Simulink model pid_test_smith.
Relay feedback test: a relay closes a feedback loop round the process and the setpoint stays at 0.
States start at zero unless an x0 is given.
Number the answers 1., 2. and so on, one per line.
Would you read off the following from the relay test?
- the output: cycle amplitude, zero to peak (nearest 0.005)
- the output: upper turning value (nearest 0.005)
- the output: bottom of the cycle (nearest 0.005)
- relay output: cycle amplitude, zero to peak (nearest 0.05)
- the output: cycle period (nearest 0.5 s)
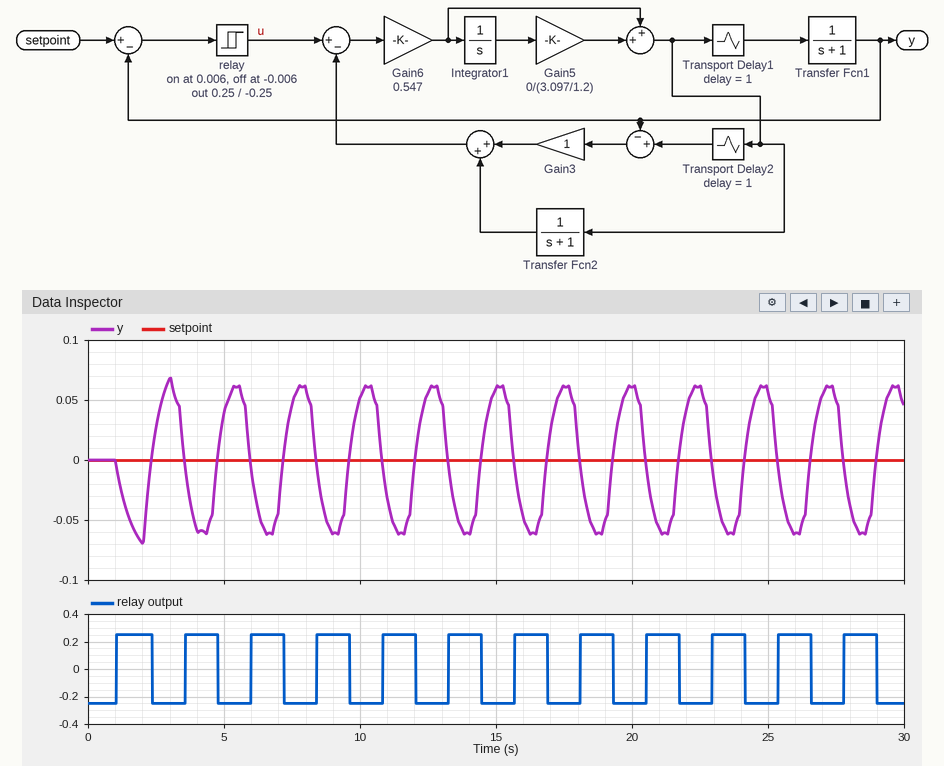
1. 0.060
2. 0.060
3. -0.060
4. 0.25
5. 2.5 s
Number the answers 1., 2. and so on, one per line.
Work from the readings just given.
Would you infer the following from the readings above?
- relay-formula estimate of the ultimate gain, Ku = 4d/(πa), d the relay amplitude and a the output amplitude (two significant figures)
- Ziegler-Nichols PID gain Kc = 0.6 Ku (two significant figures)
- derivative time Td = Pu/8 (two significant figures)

1. 5.3
2. 3.2
3. 0.31 s
